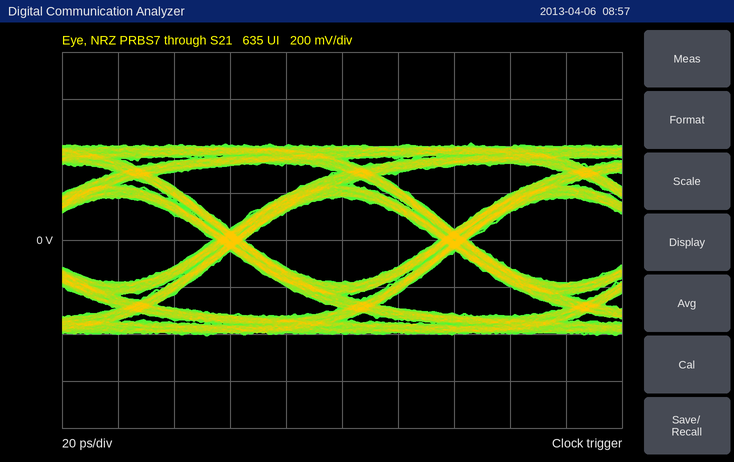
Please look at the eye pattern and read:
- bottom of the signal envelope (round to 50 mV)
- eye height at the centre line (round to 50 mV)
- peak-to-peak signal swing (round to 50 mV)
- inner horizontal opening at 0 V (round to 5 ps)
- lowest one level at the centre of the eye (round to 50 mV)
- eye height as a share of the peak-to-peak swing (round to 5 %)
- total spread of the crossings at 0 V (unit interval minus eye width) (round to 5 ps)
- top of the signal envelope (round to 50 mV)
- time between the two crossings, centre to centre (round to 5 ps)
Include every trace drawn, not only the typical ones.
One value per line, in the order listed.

-400 mV
350 mV
800 mV
70 ps
200 mV
45 %
10 ps
400 mV
80 ps
